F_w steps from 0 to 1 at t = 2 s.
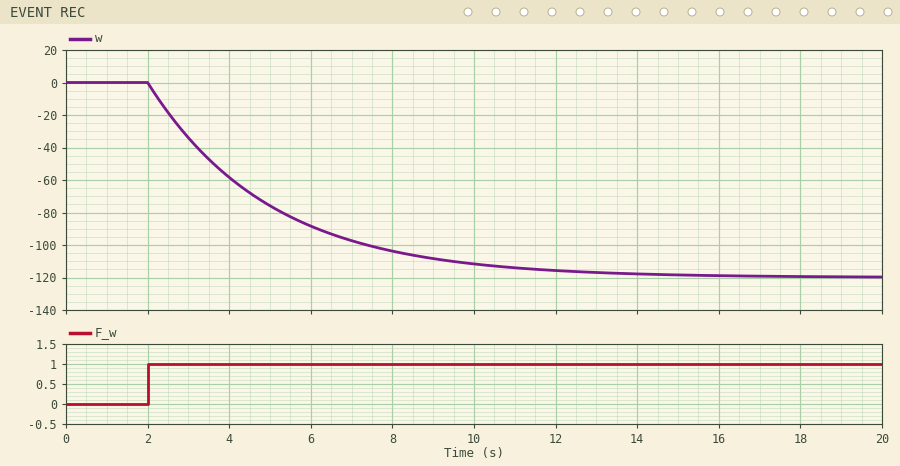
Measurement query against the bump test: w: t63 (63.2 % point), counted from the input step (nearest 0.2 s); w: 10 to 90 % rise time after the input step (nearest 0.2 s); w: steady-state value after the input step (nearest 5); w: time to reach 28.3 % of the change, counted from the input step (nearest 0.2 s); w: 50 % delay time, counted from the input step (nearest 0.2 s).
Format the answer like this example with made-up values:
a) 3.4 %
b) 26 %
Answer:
a) 3.0 s
b) 6.6 s
c) -120
d) 1.0 s
e) 2.0 s
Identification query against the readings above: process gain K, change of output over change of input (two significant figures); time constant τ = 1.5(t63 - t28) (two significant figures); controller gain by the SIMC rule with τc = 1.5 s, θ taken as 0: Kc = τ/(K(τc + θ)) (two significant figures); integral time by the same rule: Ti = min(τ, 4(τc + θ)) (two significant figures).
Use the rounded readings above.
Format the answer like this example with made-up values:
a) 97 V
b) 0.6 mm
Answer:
a) -120
b) 3.0 s
c) -0.017
d) 3.0 s
